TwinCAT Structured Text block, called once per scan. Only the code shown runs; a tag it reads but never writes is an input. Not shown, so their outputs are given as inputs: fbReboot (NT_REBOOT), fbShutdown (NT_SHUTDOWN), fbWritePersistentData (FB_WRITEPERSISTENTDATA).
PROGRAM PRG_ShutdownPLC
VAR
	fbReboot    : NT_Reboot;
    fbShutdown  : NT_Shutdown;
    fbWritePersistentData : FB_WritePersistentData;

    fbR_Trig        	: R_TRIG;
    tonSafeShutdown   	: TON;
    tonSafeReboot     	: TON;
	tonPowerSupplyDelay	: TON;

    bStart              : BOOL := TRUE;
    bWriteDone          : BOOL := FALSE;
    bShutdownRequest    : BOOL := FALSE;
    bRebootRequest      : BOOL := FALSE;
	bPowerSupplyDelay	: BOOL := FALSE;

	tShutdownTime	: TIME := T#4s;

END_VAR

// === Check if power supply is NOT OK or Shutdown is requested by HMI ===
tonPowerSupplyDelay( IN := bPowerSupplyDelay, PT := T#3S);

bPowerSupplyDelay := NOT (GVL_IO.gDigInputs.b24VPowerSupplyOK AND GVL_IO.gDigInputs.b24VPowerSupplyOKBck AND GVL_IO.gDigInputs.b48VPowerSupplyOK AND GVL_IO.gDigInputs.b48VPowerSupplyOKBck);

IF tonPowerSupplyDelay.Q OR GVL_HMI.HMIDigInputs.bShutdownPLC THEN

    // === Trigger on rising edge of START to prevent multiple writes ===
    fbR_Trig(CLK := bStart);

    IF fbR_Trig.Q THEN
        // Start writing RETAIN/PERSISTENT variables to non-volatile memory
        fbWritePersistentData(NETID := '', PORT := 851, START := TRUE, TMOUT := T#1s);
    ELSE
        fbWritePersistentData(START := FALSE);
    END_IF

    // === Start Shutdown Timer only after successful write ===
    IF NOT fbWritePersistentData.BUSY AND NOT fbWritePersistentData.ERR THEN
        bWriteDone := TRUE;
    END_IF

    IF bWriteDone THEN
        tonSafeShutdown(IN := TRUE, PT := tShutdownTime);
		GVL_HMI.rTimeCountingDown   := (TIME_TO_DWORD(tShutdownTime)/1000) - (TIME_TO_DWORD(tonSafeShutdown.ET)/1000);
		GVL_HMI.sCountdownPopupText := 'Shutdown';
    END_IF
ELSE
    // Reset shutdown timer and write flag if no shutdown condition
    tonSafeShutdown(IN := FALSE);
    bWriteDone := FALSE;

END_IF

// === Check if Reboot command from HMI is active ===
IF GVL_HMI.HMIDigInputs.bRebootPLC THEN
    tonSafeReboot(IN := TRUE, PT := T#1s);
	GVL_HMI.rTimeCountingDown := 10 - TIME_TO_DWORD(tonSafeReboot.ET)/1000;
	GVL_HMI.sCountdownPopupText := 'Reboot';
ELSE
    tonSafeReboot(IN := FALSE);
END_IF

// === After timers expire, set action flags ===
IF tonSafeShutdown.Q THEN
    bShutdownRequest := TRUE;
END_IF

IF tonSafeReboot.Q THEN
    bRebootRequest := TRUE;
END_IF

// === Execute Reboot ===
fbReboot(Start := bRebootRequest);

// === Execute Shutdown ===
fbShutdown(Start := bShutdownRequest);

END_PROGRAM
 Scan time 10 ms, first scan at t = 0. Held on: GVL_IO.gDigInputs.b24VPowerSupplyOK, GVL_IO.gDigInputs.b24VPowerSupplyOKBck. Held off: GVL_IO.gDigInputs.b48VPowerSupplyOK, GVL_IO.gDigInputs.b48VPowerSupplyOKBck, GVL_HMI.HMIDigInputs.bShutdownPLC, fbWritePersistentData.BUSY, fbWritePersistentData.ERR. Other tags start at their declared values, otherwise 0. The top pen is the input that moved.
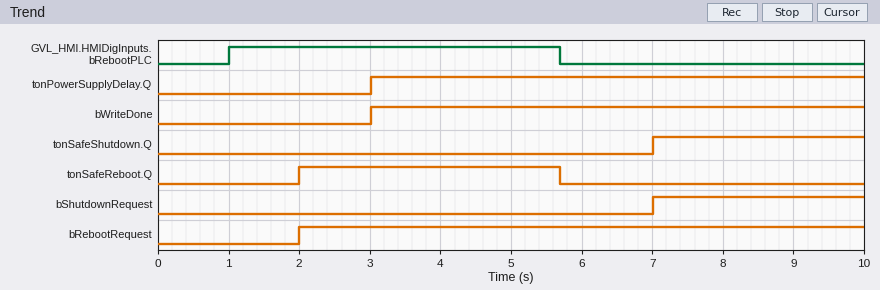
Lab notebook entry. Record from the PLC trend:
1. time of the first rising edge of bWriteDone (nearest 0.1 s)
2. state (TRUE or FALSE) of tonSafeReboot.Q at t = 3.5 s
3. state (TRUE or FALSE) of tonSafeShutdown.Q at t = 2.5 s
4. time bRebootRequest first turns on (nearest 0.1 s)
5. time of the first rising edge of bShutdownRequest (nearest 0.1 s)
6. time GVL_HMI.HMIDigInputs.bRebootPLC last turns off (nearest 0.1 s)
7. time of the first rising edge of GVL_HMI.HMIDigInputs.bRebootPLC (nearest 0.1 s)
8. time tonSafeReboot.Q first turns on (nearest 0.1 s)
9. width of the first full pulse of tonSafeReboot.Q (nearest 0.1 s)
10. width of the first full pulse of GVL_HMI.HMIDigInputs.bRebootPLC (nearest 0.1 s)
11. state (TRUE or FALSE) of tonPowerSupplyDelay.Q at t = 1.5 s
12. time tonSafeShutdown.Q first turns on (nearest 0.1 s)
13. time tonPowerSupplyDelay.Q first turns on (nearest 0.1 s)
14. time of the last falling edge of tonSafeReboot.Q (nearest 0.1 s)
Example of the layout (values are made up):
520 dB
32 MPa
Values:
3.0 s
TRUE
FALSE
2.0 s
7.0 s
5.7 s
1.0 s
2.0 s
3.7 s
4.7 s
FALSE
7.0 s
3.0 s
5.7 s
